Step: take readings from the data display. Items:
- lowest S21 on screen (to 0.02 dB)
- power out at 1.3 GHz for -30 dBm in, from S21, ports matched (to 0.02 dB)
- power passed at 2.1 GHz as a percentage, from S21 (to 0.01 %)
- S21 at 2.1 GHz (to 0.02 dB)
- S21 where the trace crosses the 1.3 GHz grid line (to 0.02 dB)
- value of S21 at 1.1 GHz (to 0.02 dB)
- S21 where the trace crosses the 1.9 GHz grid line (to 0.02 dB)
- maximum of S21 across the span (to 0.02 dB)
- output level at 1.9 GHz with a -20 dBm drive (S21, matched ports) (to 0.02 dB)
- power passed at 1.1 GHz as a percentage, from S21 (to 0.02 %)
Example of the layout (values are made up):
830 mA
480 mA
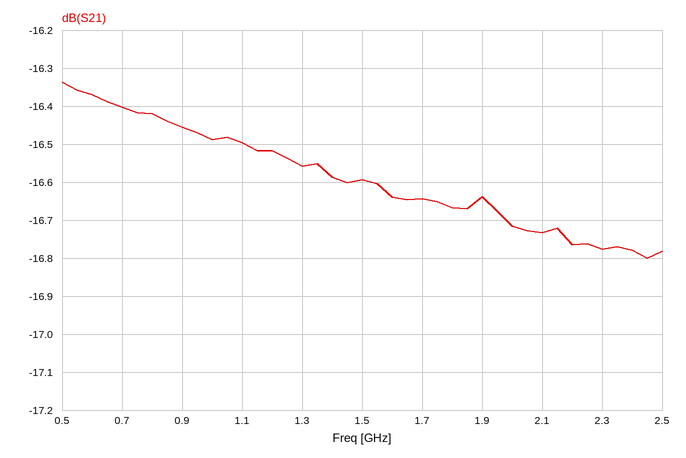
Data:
-16.80 dB
-46.56 dBm
2.12 %
-16.74 dB
-16.56 dB
-16.50 dB
-16.64 dB
-16.34 dB
-36.64 dBm
2.24 %
